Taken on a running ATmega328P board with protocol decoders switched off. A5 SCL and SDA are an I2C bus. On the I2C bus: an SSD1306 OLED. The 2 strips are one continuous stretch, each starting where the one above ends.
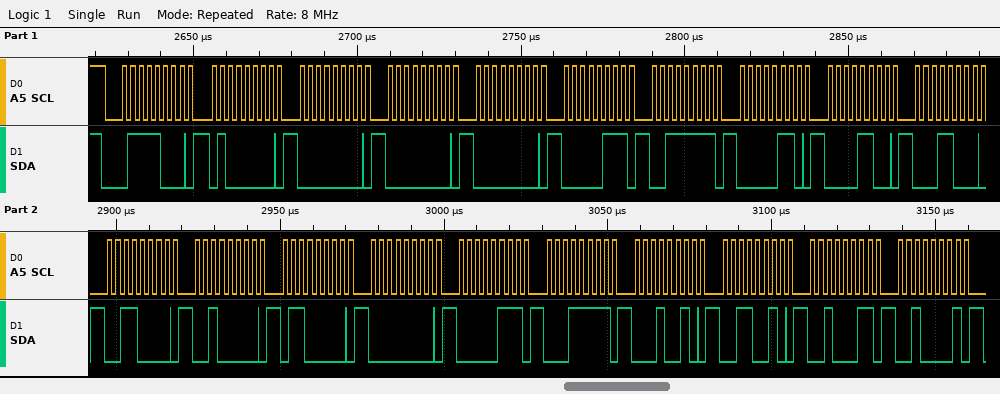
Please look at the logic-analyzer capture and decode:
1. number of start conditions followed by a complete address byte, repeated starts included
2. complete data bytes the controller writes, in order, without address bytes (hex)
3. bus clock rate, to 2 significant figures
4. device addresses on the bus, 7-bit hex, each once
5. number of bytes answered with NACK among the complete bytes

1
40 00 00 00 07 3F 06 0C 18 30 20 60 00 07 1F 12 32 23 21
400 kHz
0x3C
0
